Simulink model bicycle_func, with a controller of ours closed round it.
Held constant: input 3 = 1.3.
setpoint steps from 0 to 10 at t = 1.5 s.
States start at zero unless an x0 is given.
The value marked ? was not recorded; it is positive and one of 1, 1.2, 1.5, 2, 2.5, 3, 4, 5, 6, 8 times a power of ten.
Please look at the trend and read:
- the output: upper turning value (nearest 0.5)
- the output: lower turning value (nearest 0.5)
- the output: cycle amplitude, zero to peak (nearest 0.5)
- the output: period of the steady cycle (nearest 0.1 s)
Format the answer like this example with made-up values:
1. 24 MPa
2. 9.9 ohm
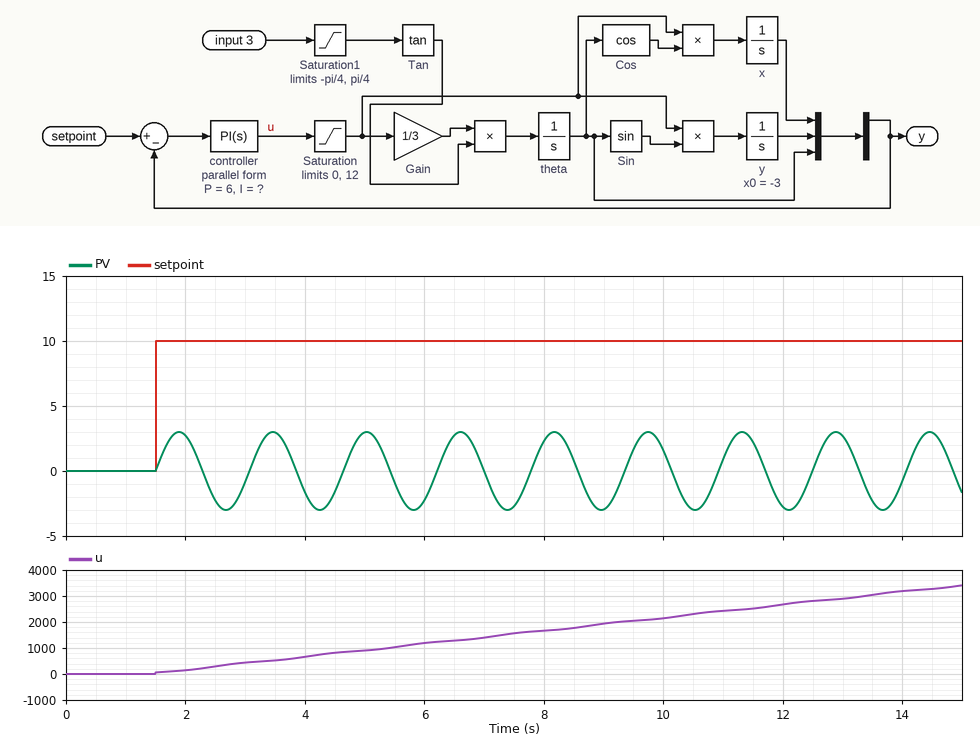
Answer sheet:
1. 3.0
2. -3.0
3. 3.0
4. 1.6 s
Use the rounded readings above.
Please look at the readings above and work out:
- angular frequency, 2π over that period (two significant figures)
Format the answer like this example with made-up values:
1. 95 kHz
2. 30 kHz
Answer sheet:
1. 3.9 rad/s
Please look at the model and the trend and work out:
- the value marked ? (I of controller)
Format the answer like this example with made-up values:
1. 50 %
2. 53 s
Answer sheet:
1. 25
